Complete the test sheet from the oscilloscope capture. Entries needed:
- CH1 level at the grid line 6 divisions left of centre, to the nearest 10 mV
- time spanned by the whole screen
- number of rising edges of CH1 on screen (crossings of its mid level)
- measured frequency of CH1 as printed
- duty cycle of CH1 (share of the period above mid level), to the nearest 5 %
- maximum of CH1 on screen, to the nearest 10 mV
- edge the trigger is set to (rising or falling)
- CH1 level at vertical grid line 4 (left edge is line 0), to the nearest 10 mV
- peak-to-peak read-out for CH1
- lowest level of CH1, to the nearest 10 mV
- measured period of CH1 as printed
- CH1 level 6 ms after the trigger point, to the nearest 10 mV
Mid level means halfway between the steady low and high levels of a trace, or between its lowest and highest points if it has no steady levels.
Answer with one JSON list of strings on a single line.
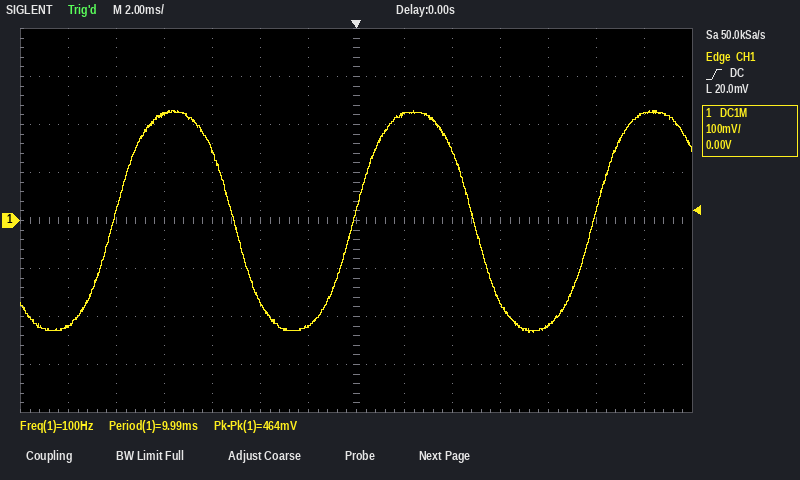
["-220 mV", "28 ms", "3", "100 Hz", "50 %", "230 mV", "rising", "150 mV", "464 mV", "-230 mV", "9.99 ms", "-170 mV"]
